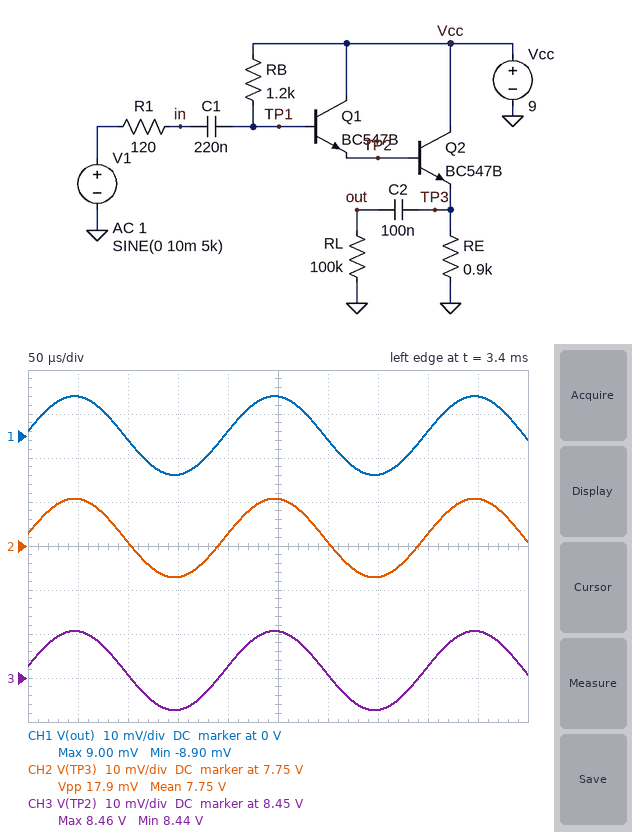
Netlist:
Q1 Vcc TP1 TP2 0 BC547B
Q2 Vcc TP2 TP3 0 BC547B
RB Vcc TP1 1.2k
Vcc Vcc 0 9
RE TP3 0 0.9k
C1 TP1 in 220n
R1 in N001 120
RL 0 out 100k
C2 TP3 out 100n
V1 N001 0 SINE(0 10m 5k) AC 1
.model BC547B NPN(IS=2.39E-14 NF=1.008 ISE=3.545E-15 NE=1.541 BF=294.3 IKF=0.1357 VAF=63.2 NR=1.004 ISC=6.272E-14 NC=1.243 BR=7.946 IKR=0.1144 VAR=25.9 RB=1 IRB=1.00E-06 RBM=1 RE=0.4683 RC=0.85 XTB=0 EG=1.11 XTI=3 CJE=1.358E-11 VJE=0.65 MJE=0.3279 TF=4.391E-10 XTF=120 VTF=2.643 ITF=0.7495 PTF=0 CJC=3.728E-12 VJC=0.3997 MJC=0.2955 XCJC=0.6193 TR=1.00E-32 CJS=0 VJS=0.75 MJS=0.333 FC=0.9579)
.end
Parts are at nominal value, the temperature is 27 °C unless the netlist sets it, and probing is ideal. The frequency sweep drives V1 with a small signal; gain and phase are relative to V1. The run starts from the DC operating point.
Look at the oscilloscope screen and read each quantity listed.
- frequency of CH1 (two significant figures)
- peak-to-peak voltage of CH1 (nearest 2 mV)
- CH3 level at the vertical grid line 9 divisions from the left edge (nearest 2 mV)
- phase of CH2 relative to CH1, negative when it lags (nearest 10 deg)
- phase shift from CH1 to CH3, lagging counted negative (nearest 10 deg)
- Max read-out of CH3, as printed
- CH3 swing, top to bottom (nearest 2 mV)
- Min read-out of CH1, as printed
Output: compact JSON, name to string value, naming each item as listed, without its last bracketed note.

{"frequency of CH1": "5.0 kHz", "peak-to-peak voltage of CH1": "18 mV", "CH3 level at the vertical grid line 9 divisions from the left edge": "8.460 V", "phase of CH2 relative to CH1, negative when it lags": "0 deg", "phase shift from CH1 to CH3, lagging counted negative": "0 deg", "Max read-out of CH3, as printed": "8.46 V", "CH3 swing, top to bottom": "18 mV", "Min read-out of CH1, as printed": "-8.90 mV"}
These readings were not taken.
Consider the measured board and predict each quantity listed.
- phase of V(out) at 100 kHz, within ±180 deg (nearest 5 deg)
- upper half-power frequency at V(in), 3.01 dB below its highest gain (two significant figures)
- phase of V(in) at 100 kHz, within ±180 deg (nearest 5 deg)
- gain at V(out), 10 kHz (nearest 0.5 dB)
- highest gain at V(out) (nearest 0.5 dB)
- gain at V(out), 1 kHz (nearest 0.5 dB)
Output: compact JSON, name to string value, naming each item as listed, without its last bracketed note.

{"phase of V(out) at 100 kHz, within ±180 deg": "0 deg", "upper half-power frequency at V(in), 3.01 dB below its highest gain": "170 MHz", "phase of V(in) at 100 kHz, within ±180 deg": "0 deg", "gain at V(out), 10 kHz": "-1.0 dB", "highest gain at V(out)": "-1.0 dB", "gain at V(out), 1 kHz": "-2.0 dB"}
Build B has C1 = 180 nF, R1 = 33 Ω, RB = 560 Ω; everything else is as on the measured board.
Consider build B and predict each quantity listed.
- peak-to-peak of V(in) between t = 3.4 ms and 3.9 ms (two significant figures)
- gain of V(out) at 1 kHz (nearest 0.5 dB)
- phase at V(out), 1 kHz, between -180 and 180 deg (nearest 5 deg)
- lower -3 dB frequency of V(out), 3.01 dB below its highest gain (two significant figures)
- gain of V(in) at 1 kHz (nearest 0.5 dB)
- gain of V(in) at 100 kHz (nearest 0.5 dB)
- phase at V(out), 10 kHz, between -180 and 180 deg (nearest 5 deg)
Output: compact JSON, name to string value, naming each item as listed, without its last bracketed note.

{"peak-to-peak of V(in) between t = 3.4 ms and 3.9 ms": "19 mV", "gain of V(out) at 1 kHz": "-5.5 dB", "phase at V(out), 1 kHz, between -180 and 180 deg": "55 deg", "lower -3 dB frequency of V(out), 3.01 dB below its highest gain": "1.5 kHz", "gain of V(in) at 1 kHz": "0 dB", "gain of V(in) at 100 kHz": "-0.5 dB", "phase at V(out), 10 kHz, between -180 and 180 deg": "10 deg"}
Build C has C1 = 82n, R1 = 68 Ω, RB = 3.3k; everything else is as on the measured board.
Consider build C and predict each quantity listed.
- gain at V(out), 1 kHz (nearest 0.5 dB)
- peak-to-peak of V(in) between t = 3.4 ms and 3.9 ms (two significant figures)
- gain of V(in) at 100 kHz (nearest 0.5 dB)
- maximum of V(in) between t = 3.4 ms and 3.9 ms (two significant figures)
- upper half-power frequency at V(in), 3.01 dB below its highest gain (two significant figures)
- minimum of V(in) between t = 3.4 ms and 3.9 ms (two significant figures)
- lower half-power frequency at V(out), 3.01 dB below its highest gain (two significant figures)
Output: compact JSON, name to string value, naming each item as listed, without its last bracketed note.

{"gain at V(out), 1 kHz": "-1.5 dB", "peak-to-peak of V(in) between t = 3.4 ms and 3.9 ms": "20 mV", "gain of V(in) at 100 kHz": "0 dB", "maximum of V(in) between t = 3.4 ms and 3.9 ms": "9.8 mV", "upper half-power frequency at V(in), 3.01 dB below its highest gain": "330 MHz", "minimum of V(in) between t = 3.4 ms and 3.9 ms": "-9.8 mV", "lower half-power frequency at V(out), 3.01 dB below its highest gain": "580 Hz"}
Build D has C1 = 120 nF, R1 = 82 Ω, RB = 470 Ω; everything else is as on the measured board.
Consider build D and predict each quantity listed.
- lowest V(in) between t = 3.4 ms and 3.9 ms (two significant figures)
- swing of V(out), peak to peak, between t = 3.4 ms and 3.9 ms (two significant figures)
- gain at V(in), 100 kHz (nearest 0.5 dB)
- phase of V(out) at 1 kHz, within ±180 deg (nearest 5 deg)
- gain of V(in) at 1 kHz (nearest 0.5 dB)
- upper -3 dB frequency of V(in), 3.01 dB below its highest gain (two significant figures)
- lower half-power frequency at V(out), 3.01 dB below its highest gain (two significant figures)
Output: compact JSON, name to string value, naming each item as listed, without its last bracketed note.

{"lowest V(in) between t = 3.4 ms and 3.9 ms": "-8.8 mV", "swing of V(out), peak to peak, between t = 3.4 ms and 3.9 ms": "15 mV", "gain at V(in), 100 kHz": "-1.5 dB", "phase of V(out) at 1 kHz, within ±180 deg": "70 deg", "gain of V(in) at 1 kHz": "0 dB", "upper -3 dB frequency of V(in), 3.01 dB below its highest gain": "210 MHz", "lower half-power frequency at V(out), 3.01 dB below its highest gain": "2.4 kHz"}
